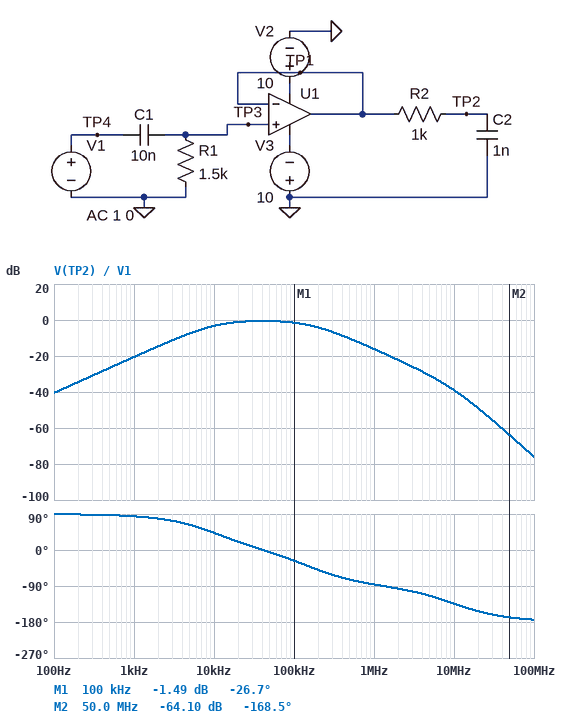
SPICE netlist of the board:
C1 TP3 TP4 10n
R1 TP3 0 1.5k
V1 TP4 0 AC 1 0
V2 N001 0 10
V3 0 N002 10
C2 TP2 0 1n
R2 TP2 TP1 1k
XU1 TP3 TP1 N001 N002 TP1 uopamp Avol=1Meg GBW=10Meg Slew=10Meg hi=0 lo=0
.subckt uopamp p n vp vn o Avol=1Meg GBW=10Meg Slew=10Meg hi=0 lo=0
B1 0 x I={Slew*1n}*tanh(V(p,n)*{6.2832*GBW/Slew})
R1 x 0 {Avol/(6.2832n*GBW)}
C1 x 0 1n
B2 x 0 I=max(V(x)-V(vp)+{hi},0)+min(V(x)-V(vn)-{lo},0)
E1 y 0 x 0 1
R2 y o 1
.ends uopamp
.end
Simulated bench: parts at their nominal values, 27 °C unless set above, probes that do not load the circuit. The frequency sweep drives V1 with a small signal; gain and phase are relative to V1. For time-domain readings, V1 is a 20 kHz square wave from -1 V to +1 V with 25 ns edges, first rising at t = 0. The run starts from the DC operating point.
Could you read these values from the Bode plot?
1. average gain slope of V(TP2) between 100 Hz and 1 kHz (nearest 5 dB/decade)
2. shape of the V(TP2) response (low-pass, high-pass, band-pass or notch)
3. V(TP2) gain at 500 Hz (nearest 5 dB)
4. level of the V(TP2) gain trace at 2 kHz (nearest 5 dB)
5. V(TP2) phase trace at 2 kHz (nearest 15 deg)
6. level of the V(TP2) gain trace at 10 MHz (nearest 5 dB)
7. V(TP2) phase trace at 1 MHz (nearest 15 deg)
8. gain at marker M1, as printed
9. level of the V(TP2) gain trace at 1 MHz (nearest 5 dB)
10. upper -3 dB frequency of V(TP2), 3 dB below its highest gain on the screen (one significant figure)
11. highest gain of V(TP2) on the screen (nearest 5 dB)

20 dB/decade
band-pass
-25 dB
-15 dB
75 deg
-40 dB
-90 deg
-1.49 dB
-15 dB
200 kHz
0 dB
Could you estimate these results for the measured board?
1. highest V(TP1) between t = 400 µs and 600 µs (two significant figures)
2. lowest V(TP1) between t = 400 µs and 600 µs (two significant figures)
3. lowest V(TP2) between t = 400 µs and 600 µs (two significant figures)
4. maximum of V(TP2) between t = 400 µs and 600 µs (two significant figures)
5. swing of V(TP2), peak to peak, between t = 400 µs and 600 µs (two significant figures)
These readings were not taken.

1.7 V
-1.7 V
-1.4 V
1.4 V
2.7 V
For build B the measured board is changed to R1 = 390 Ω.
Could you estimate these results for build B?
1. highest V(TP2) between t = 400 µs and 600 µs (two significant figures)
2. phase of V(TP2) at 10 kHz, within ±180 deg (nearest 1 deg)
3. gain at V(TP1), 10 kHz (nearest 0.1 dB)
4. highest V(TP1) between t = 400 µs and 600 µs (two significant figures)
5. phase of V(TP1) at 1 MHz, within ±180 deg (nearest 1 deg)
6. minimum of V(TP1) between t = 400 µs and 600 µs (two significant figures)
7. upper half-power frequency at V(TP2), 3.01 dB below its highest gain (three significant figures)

1.2 V
73 deg
-12.5 dB
1.9 V
-3 deg
-1.9 V
228 kHz
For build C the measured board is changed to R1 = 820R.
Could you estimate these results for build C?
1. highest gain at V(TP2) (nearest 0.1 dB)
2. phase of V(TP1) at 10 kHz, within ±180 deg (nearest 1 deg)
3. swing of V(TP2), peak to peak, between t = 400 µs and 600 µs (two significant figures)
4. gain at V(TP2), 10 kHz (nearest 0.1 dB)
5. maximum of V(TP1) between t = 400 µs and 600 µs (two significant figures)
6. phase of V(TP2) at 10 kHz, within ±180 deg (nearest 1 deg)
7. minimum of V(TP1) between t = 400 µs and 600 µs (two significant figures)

-1.0 dB
63 deg
2.8 V
-6.8 dB
1.9 V
59 deg
-1.9 V
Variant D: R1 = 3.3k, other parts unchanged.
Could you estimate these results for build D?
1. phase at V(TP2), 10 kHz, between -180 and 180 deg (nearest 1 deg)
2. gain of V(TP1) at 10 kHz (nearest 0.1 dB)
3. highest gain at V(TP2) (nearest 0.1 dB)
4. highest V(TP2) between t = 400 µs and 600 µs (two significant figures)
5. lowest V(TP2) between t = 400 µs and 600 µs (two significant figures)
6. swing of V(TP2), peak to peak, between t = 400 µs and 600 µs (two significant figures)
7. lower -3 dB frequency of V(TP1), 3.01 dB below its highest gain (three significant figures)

22 deg
-0.9 dB
-0.3 dB
1.2 V
-1.2 V
2.4 V
4.82 kHz
